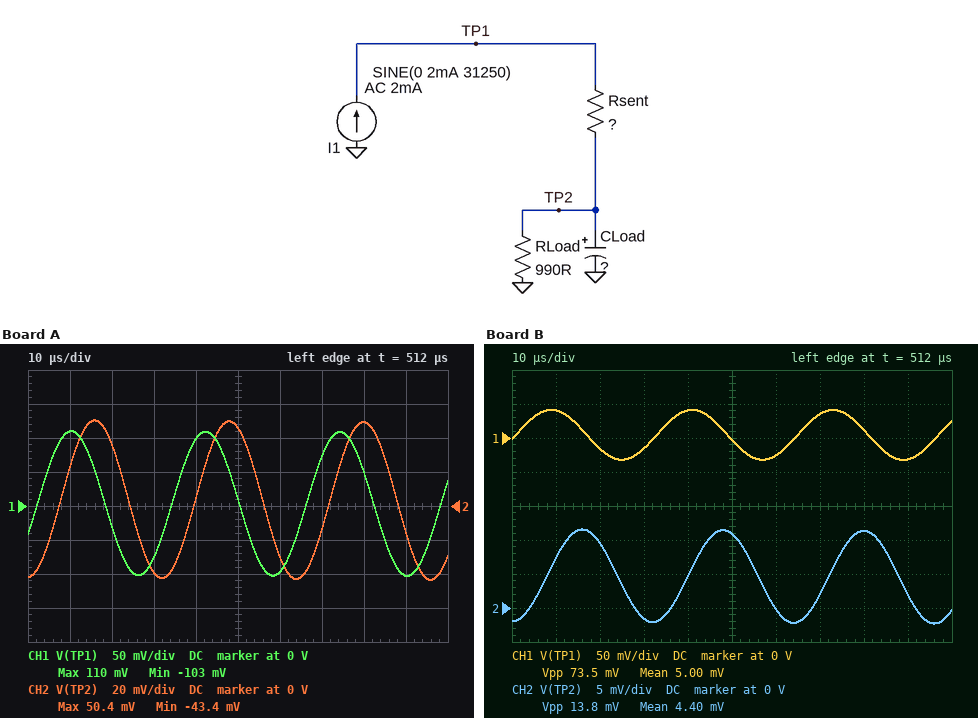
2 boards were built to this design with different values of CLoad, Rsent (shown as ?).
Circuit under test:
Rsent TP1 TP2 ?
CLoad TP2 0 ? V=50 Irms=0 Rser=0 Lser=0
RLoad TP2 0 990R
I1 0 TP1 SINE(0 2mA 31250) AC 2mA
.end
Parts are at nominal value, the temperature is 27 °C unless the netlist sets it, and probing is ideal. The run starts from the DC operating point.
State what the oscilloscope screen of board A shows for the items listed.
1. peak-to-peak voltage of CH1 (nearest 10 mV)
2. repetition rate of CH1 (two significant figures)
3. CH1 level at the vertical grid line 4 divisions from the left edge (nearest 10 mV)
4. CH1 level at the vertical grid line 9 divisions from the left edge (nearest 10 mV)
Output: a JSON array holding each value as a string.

["210 mV", "31 kHz", "100 mV", "-100 mV"]
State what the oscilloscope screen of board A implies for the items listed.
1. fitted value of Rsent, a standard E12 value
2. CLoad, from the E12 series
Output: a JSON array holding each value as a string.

["47 Ω", "220 nF"]
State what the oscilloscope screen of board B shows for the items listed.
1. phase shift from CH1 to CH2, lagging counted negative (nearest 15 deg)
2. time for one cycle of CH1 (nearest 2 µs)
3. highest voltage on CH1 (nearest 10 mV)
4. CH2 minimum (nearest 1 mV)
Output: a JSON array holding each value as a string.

["-75 deg", "32 µs", "40 mV", "-2 mV"]
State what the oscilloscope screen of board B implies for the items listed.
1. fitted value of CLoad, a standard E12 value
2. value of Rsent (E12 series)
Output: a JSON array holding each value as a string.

["1.5 µF", "18 Ω"]
